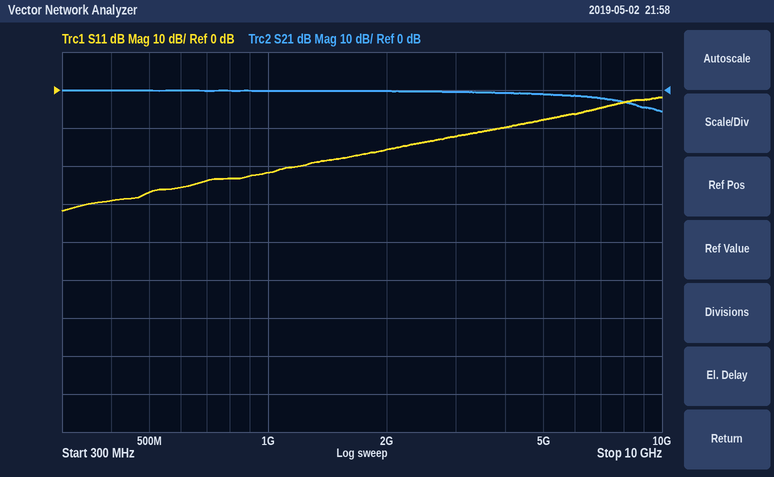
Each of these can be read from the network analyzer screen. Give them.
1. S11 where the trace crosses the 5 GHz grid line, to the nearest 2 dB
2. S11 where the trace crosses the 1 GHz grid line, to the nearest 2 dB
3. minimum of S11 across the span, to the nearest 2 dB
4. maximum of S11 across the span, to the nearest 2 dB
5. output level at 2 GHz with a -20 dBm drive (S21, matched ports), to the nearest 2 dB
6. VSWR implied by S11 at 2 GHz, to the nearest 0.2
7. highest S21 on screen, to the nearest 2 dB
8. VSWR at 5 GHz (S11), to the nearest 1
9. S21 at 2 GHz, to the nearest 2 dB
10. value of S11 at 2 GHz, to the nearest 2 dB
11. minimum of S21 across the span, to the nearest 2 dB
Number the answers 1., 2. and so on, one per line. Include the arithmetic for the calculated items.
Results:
1. -8 dB
2. -22 dB
3. -32 dB
4. -2 dB
5. -20 dBm + (0 dB) = -20 dBm
6. |Γ| = 10^(-16/20) = 0.1585; VSWR = (1 + 0.1585)/(1 − 0.1585) ≈ 1.4
7. 0 dB
8. |Γ| = 10^(-8/20) = 0.3981; VSWR = (1 + 0.3981)/(1 − 0.3981) ≈ 2
9. 0 dB
10. -16 dB
11. -6 dB
